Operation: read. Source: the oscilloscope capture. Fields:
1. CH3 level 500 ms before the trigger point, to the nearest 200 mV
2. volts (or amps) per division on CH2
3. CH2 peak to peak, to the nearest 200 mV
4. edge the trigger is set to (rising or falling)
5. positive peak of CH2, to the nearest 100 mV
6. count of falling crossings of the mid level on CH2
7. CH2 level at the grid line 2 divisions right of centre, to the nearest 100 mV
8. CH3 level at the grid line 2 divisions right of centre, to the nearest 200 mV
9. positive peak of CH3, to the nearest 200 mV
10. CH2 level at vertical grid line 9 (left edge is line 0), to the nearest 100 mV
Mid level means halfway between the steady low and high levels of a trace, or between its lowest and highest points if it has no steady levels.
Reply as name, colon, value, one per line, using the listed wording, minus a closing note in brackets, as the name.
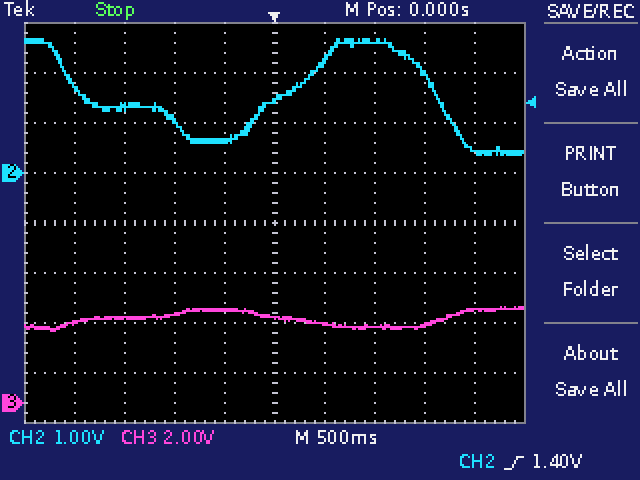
CH3 level 500 ms before the trigger point, to the nearest 200 mV: 3.8 V
volts (or amps) per division on CH2: 1 V
CH2 peak to peak, to the nearest 200 mV: 2.4 V
edge the trigger is set to: rising
positive peak of CH2, to the nearest 100 mV: 2.7 V
count of falling crossings of the mid level on CH2: 2
CH2 level at the grid line 2 divisions right of centre, to the nearest 100 mV: 2.6 V
CH3 level at the grid line 2 divisions right of centre, to the nearest 200 mV: 3.0 V
positive peak of CH3, to the nearest 200 mV: 3.8 V
CH2 level at vertical grid line 9 (left edge is line 0), to the nearest 100 mV: 400 mV
